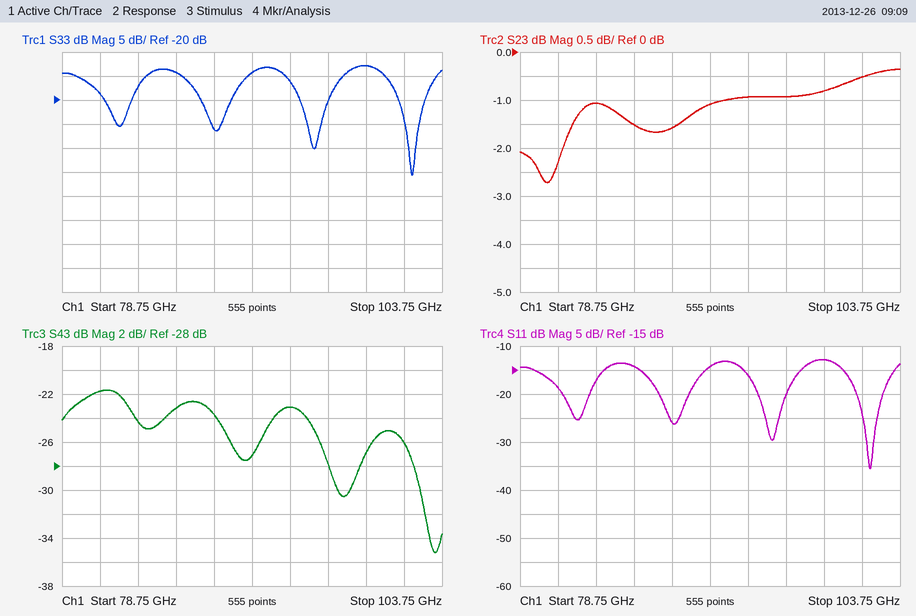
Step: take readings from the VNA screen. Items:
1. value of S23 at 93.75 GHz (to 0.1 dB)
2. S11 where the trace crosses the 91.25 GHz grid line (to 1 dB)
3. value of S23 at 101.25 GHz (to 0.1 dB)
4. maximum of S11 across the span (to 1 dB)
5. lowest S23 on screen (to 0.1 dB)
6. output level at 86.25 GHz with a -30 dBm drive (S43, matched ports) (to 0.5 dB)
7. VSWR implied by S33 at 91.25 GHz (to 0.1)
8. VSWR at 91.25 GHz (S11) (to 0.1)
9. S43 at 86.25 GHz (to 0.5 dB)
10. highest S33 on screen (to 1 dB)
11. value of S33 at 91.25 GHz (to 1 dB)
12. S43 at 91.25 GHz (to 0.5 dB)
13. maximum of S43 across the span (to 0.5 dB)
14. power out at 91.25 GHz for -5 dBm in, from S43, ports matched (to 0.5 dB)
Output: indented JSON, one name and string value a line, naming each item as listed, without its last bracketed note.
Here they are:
{
  "value of S23 at 93.75 GHz": "-0.9 dB",
  "S11 where the trace crosses the 91.25 GHz grid line": "-14 dB",
  "value of S23 at 101.25 GHz": "-0.5 dB",
  "maximum of S11 across the span": "-13 dB",
  "lowest S23 on screen": "-2.7 dB",
  "output level at 86.25 GHz with a -30 dBm drive (S43, matched ports)": "-53.0 dBm",
  "VSWR implied by S33 at 91.25 GHz": "1.5",
  "VSWR at 91.25 GHz (S11)": "1.5",
  "S43 at 86.25 GHz": "-23.0 dB",
  "highest S33 on screen": "-13 dB",
  "value of S33 at 91.25 GHz": "-14 dB",
  "S43 at 91.25 GHz": "-27.0 dB",
  "maximum of S43 across the span": "-21.5 dB",
  "power out at 91.25 GHz for -5 dBm in, from S43, ports matched": "-32.0 dBm"
}
